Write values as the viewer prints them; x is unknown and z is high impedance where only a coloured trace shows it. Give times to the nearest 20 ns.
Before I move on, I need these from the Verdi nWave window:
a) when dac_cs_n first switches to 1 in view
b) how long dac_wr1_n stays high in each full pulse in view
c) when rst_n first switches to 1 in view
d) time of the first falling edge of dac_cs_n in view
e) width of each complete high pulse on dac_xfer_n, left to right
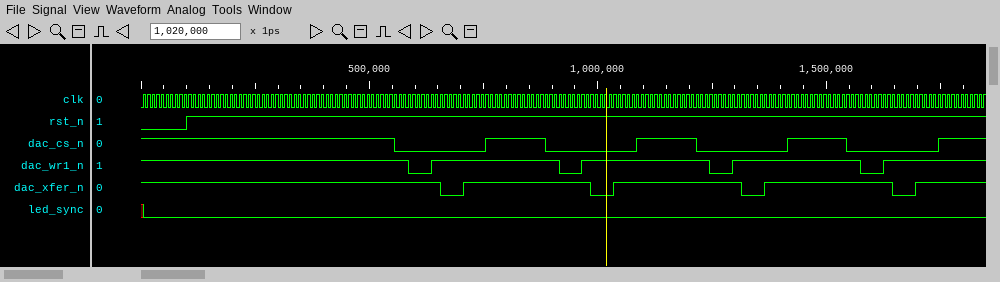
760 ns
280 ns, 280 ns, 280 ns
100 ns
560 ns
280 ns, 280 ns, 280 ns
